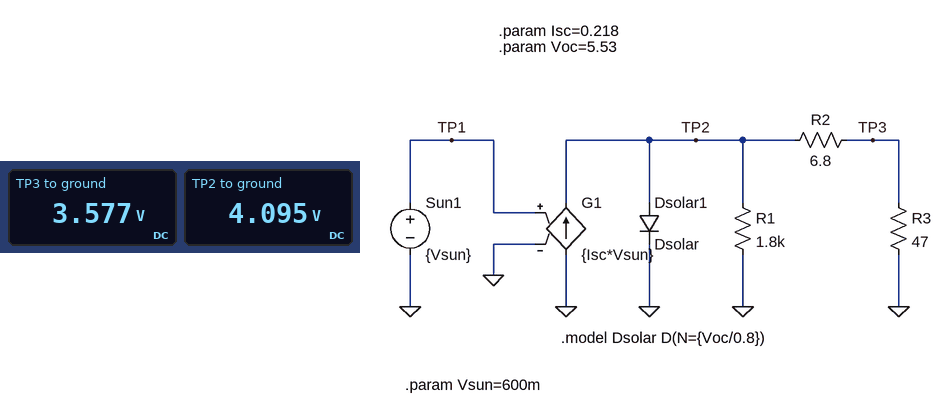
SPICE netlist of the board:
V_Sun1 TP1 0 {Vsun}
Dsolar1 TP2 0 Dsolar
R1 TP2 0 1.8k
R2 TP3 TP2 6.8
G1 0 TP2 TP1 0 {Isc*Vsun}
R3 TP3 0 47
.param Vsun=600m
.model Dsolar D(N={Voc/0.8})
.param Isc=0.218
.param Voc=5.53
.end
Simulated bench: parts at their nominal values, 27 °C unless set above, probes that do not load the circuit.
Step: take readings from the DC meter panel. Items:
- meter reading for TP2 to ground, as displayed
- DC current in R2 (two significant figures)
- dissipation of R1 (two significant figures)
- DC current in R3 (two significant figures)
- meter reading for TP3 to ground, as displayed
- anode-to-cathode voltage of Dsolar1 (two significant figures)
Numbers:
4.095 V
76 mA
9.3 mW
76 mA
3.577 V
4.1 V
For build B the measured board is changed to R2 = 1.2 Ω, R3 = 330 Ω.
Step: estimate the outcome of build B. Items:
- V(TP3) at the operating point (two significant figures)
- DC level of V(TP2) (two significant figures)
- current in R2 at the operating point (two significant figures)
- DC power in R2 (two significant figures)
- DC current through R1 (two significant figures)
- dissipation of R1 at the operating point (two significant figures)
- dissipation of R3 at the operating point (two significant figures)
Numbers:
5.2 V
5.3 V
16 mA
300 µW
2.9 mA
15 mW
83 mW
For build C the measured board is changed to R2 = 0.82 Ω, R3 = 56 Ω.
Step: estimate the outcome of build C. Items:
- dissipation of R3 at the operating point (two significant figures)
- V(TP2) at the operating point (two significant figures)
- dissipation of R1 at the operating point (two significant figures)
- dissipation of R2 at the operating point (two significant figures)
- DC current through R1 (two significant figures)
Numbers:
320 mW
4.3 V
10 mW
4.7 mW
2.4 mA
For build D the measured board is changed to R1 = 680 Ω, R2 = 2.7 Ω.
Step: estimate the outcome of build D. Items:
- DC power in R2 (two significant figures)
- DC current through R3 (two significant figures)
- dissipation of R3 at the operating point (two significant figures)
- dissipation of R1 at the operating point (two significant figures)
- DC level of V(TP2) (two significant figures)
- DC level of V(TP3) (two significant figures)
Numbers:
14 mW
73 mA
250 mW
19 mW
3.6 V
3.4 V
